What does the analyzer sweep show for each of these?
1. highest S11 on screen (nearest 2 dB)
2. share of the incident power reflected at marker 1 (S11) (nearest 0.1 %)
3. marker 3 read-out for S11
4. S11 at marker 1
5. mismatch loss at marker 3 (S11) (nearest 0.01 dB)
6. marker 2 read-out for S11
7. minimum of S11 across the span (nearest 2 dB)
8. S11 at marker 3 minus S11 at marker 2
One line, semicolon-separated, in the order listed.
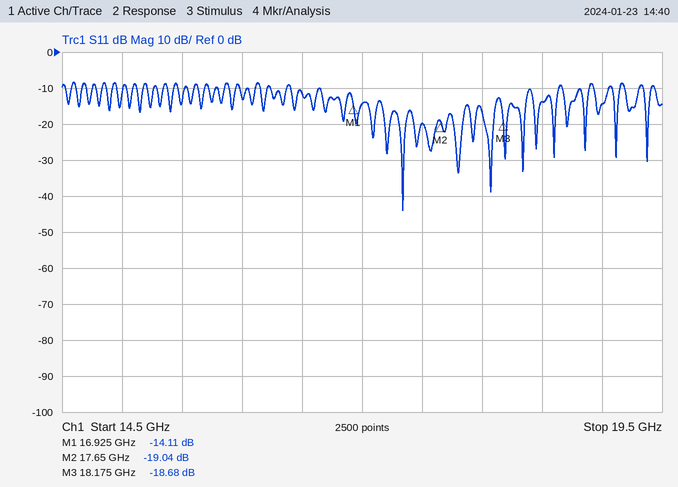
-8 dB; 3.9 %; -18.68 dB; -14.11 dB; 0.06 dB; -19.04 dB; -44 dB; 0.36 dB
